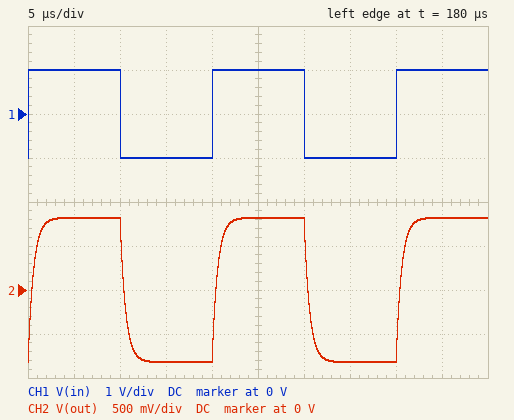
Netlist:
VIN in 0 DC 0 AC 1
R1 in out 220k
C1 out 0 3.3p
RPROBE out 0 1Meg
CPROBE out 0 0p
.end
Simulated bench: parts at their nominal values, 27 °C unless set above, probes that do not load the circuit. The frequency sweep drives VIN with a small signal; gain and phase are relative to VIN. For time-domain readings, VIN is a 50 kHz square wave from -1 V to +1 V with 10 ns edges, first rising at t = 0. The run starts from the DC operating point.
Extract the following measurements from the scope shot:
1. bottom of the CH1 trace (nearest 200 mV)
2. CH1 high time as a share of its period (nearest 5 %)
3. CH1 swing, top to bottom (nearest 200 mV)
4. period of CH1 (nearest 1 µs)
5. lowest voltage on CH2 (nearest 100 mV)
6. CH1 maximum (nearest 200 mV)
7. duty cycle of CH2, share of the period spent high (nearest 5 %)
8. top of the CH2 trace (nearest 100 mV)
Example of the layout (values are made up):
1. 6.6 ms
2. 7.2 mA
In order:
1. -1.0 V
2. 50 %
3. 2.0 V
4. 20 µs
5. -800 mV
6. 1.0 V
7. 50 %
8. 800 mV
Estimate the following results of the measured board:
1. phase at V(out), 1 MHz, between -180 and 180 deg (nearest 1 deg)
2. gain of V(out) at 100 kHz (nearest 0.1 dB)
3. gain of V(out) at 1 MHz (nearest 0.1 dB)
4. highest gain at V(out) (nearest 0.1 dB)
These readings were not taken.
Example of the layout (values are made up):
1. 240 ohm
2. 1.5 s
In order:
1. -75 deg
2. -2.3 dB
3. -13.5 dB
4. -1.7 dB
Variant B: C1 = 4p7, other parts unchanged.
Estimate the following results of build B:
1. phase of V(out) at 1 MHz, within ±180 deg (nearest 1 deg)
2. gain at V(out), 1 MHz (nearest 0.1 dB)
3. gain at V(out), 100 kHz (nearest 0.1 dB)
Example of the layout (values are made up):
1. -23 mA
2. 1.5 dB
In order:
1. -79 deg
2. -16.4 dB
3. -2.8 dB
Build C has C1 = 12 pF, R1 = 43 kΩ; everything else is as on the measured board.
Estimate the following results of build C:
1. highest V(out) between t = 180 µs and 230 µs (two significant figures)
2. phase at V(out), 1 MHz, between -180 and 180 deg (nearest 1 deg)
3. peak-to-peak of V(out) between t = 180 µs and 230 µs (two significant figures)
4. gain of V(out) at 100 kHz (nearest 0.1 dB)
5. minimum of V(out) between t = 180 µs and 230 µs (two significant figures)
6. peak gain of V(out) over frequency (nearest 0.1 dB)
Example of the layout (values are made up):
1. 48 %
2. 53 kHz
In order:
1. 960 mV
2. -72 deg
3. 1.9 V
4. -0.8 dB
5. -960 mV
6. -0.4 dB
